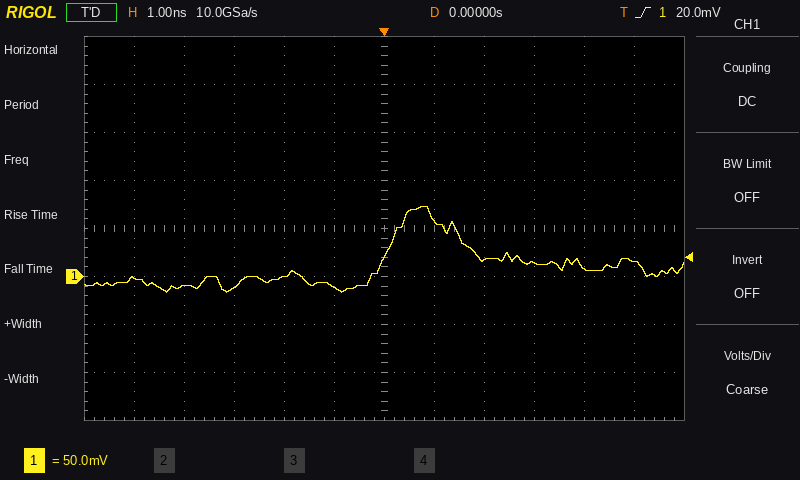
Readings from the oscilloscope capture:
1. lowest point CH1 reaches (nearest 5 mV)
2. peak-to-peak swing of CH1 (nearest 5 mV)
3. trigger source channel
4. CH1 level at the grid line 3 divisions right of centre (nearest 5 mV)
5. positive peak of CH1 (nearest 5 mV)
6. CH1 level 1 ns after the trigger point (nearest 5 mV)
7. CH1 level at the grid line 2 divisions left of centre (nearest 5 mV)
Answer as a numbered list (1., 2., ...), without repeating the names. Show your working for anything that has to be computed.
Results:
1. -15 mV
2. 75 mV − (-15 mV) = 90 mV
3. CH1
4. 15 mV
5. 75 mV
6. 60 mV
7. 0 mV
